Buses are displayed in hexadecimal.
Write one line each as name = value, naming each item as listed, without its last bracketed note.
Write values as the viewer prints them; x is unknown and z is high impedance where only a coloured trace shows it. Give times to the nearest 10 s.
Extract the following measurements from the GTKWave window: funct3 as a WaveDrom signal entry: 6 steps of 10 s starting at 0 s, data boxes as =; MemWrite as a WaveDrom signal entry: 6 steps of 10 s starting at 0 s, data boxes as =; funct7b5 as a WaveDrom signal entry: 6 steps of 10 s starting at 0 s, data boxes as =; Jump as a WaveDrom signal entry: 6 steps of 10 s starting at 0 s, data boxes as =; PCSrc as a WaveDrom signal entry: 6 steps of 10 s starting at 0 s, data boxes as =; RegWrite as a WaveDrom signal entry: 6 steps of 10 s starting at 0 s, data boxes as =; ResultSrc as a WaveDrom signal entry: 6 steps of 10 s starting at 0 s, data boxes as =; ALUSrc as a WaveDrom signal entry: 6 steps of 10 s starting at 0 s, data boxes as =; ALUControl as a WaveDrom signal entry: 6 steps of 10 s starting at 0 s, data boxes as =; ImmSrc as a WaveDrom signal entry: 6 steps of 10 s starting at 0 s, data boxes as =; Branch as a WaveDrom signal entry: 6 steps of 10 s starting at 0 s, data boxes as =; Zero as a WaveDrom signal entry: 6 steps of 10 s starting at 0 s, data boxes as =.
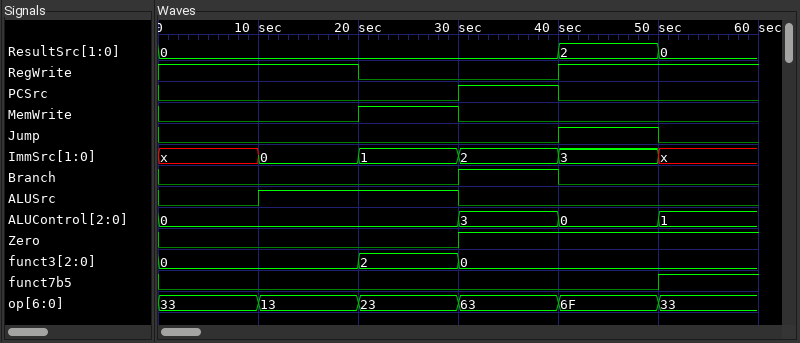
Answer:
funct3 as a WaveDrom signal entry: 6 steps of 10 s starting at 0 s, data boxes as = = {name: 'funct3', wave: '=.==..', data: '0 2 0'}
MemWrite as a WaveDrom signal entry: 6 steps of 10 s starting at 0 s, data boxes as = = {name: 'MemWrite', wave: '0.10..'}
funct7b5 as a WaveDrom signal entry: 6 steps of 10 s starting at 0 s, data boxes as = = {name: 'funct7b5', wave: '0....1'}
Jump as a WaveDrom signal entry: 6 steps of 10 s starting at 0 s, data boxes as = = {name: 'Jump', wave: '0...10'}
PCSrc as a WaveDrom signal entry: 6 steps of 10 s starting at 0 s, data boxes as = = {name: 'PCSrc', wave: '0..10.'}
RegWrite as a WaveDrom signal entry: 6 steps of 10 s starting at 0 s, data boxes as = = {name: 'RegWrite', wave: '1.0.1.'}
ResultSrc as a WaveDrom signal entry: 6 steps of 10 s starting at 0 s, data boxes as = = {name: 'ResultSrc', wave: '=...==', data: '0 2 0'}
ALUSrc as a WaveDrom signal entry: 6 steps of 10 s starting at 0 s, data boxes as = = {name: 'ALUSrc', wave: '01.0..'}
ALUControl as a WaveDrom signal entry: 6 steps of 10 s starting at 0 s, data boxes as = = {name: 'ALUControl', wave: '=..===', data: '0 3 0 1'}
ImmSrc as a WaveDrom signal entry: 6 steps of 10 s starting at 0 s, data boxes as = = {name: 'ImmSrc', wave: 'x====x', data: '0 1 2 3'}
Branch as a WaveDrom signal entry: 6 steps of 10 s starting at 0 s, data boxes as = = {name: 'Branch', wave: '0..10.'}
Zero as a WaveDrom signal entry: 6 steps of 10 s starting at 0 s, data boxes as = = {name: 'Zero', wave: '0..1..'}
